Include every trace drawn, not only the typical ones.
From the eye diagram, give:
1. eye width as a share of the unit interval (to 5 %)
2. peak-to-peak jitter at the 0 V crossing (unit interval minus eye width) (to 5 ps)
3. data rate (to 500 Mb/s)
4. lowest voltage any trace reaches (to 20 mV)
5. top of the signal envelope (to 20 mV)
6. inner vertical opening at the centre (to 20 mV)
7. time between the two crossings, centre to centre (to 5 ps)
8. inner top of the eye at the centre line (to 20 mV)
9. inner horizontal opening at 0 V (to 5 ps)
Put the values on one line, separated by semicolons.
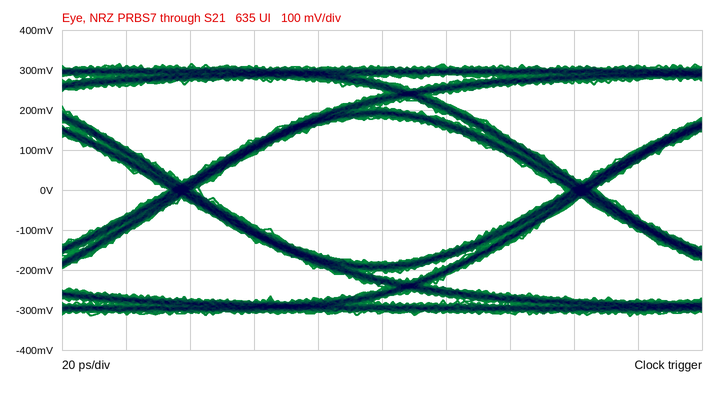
90 %; 10 ps; 8.0 Gb/s; -320 mV; 320 mV; 360 mV; 125 ps; 180 mV; 115 ps
